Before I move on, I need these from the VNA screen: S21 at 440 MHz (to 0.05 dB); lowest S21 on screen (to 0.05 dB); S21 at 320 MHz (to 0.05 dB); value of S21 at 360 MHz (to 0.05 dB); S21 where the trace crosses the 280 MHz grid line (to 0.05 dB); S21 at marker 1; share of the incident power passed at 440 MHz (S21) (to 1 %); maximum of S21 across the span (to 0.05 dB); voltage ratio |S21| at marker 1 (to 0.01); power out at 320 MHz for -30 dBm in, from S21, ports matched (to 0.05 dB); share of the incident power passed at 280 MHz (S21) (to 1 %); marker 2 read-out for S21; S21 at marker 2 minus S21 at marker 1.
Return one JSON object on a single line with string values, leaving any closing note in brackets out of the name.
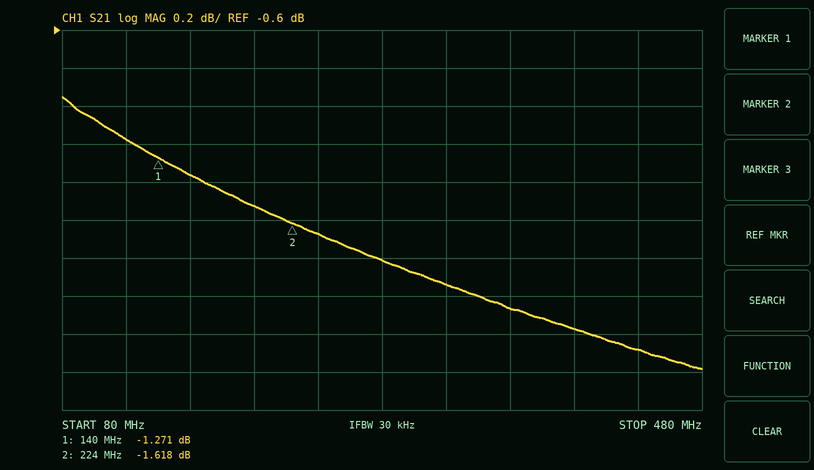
{"S21 at 440 MHz": "-2.30 dB", "lowest S21 on screen": "-2.40 dB", "S21 at 320 MHz": "-1.95 dB", "value of S21 at 360 MHz": "-2.05 dB", "S21 where the trace crosses the 280 MHz grid line": "-1.80 dB", "S21 at marker 1": "-1.271 dB", "share of the incident power passed at 440 MHz (S21)": "59 %", "maximum of S21 across the span": "-0.95 dB", "voltage ratio |S21| at marker 1": "0.86", "power out at 320 MHz for -30 dBm in, from S21, ports matched": "-31.95 dBm", "share of the incident power passed at 280 MHz (S21)": "66 %", "marker 2 read-out for S21": "-1.618 dB", "S21 at marker 2 minus S21 at marker 1": "-0.347 dB"}
